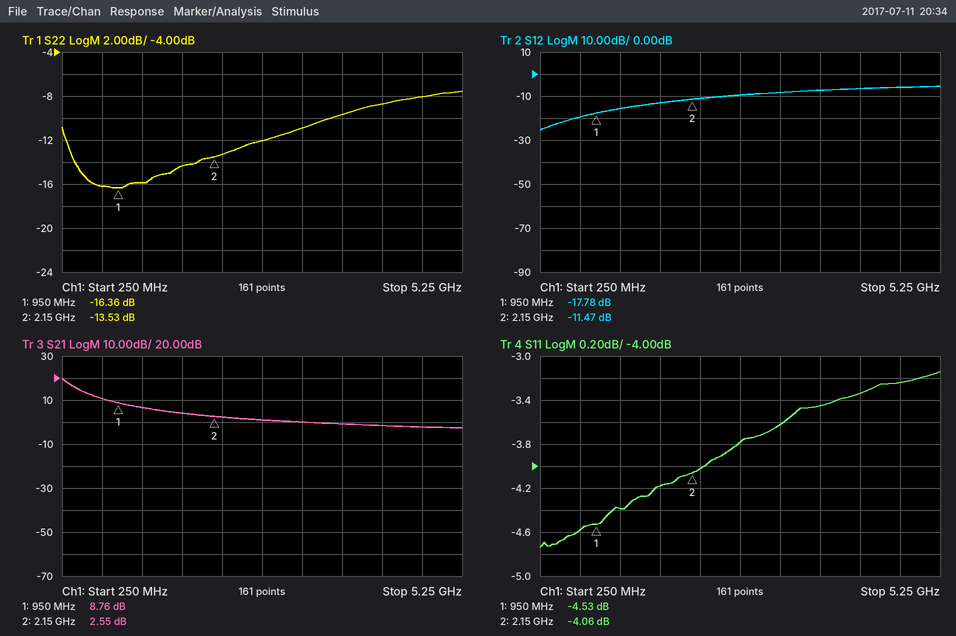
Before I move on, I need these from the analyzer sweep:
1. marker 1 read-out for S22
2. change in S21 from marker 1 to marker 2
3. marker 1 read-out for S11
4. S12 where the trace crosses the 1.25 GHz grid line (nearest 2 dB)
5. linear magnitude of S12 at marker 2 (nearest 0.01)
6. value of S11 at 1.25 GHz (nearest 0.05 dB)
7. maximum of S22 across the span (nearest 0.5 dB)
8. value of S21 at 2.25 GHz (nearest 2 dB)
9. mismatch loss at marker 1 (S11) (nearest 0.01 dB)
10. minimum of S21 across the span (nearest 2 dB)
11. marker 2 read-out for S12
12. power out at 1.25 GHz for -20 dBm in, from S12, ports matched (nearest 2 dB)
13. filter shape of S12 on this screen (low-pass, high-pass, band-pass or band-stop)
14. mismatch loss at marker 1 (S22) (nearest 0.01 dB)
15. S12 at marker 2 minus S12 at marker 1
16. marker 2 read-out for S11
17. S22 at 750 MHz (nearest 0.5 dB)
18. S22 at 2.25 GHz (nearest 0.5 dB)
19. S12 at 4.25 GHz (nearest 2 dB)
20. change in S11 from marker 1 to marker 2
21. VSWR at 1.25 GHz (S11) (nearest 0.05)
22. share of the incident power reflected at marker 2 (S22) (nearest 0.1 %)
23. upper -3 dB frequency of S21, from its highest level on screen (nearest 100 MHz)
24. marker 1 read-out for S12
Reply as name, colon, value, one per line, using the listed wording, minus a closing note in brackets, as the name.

marker 1 read-out for S22: -16.36 dB
change in S21 from marker 1 to marker 2: -6.21 dB
marker 1 read-out for S11: -4.53 dB
S12 where the trace crosses the 1.25 GHz grid line: -16 dB
linear magnitude of S12 at marker 2: 0.27
value of S11 at 1.25 GHz: -4.40 dB
maximum of S22 across the span: -7.5 dB
value of S21 at 2.25 GHz: 2 dB
mismatch loss at marker 1 (S11): 1.89 dB
minimum of S21 across the span: -2 dB
marker 2 read-out for S12: -11.47 dB
power out at 1.25 GHz for -20 dBm in, from S12, ports matched: -36 dBm
filter shape of S12 on this screen: high-pass
mismatch loss at marker 1 (S22): 0.10 dB
S12 at marker 2 minus S12 at marker 1: 6.31 dB
marker 2 read-out for S11: -4.06 dB
S22 at 750 MHz: -16.0 dB
S22 at 2.25 GHz: -13.5 dB
S12 at 4.25 GHz: -6 dB
change in S11 from marker 1 to marker 2: 0.47 dB
VSWR at 1.25 GHz (S11): 4.05
share of the incident power reflected at marker 2 (S22): 4.4 %
upper -3 dB frequency of S21, from its highest level on screen: 400 MHz
marker 1 read-out for S12: -17.78 dB
